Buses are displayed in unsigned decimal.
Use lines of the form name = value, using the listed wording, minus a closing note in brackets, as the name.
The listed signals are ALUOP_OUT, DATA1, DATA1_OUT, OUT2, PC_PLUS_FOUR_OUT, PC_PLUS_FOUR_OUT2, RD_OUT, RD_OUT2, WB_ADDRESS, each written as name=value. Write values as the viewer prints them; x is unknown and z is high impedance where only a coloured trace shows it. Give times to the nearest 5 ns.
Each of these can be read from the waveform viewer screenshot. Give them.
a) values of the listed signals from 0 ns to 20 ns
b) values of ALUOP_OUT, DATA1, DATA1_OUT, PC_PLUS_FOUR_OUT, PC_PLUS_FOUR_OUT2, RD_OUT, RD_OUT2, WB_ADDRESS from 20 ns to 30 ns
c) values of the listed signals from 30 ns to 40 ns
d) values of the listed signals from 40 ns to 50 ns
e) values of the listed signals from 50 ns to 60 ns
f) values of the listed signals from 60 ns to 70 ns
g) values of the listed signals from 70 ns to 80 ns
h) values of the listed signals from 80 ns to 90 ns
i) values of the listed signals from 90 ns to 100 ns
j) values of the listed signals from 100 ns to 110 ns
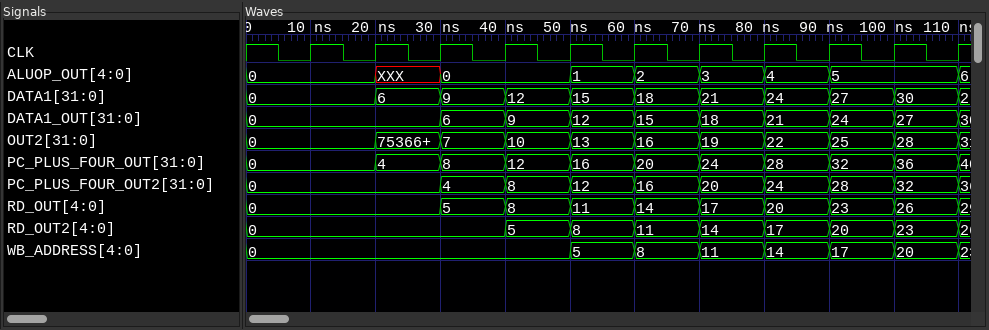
values of the listed signals from 0 ns to 20 ns = ALUOP_OUT=0, DATA1=0, DATA1_OUT=0, OUT2=0, PC_PLUS_FOUR_OUT=0, PC_PLUS_FOUR_OUT2=0, RD_OUT=0, RD_OUT2=0, WB_ADDRESS=0
values of ALUOP_OUT, DATA1, DATA1_OUT, PC_PLUS_FOUR_OUT, PC_PLUS_FOUR_OUT2, RD_OUT, RD_OUT2, WB_ADDRESS from 20 ns to 30 ns = ALUOP_OUT=XXX, DATA1=6, DATA1_OUT=0, PC_PLUS_FOUR_OUT=4, PC_PLUS_FOUR_OUT2=0, RD_OUT=0, RD_OUT2=0, WB_ADDRESS=0
values of the listed signals from 30 ns to 40 ns = ALUOP_OUT=0, DATA1=9, DATA1_OUT=6, OUT2=7, PC_PLUS_FOUR_OUT=8, PC_PLUS_FOUR_OUT2=4, RD_OUT=5, RD_OUT2=0, WB_ADDRESS=0
values of the listed signals from 40 ns to 50 ns = ALUOP_OUT=0, DATA1=12, DATA1_OUT=9, OUT2=10, PC_PLUS_FOUR_OUT=12, PC_PLUS_FOUR_OUT2=8, RD_OUT=8, RD_OUT2=5, WB_ADDRESS=0
values of the listed signals from 50 ns to 60 ns = ALUOP_OUT=1, DATA1=15, DATA1_OUT=12, OUT2=13, PC_PLUS_FOUR_OUT=16, PC_PLUS_FOUR_OUT2=12, RD_OUT=11, RD_OUT2=8, WB_ADDRESS=5
values of the listed signals from 60 ns to 70 ns = ALUOP_OUT=2, DATA1=18, DATA1_OUT=15, OUT2=16, PC_PLUS_FOUR_OUT=20, PC_PLUS_FOUR_OUT2=16, RD_OUT=14, RD_OUT2=11, WB_ADDRESS=8
values of the listed signals from 70 ns to 80 ns = ALUOP_OUT=3, DATA1=21, DATA1_OUT=18, OUT2=19, PC_PLUS_FOUR_OUT=24, PC_PLUS_FOUR_OUT2=20, RD_OUT=17, RD_OUT2=14, WB_ADDRESS=11
values of the listed signals from 80 ns to 90 ns = ALUOP_OUT=4, DATA1=24, DATA1_OUT=21, OUT2=22, PC_PLUS_FOUR_OUT=28, PC_PLUS_FOUR_OUT2=24, RD_OUT=20, RD_OUT2=17, WB_ADDRESS=14
values of the listed signals from 90 ns to 100 ns = ALUOP_OUT=5, DATA1=27, DATA1_OUT=24, OUT2=25, PC_PLUS_FOUR_OUT=32, PC_PLUS_FOUR_OUT2=28, RD_OUT=23, RD_OUT2=20, WB_ADDRESS=17
values of the listed signals from 100 ns to 110 ns = ALUOP_OUT=5, DATA1=30, DATA1_OUT=27, OUT2=28, PC_PLUS_FOUR_OUT=36, PC_PLUS_FOUR_OUT2=32, RD_OUT=26, RD_OUT2=23, WB_ADDRESS=20
